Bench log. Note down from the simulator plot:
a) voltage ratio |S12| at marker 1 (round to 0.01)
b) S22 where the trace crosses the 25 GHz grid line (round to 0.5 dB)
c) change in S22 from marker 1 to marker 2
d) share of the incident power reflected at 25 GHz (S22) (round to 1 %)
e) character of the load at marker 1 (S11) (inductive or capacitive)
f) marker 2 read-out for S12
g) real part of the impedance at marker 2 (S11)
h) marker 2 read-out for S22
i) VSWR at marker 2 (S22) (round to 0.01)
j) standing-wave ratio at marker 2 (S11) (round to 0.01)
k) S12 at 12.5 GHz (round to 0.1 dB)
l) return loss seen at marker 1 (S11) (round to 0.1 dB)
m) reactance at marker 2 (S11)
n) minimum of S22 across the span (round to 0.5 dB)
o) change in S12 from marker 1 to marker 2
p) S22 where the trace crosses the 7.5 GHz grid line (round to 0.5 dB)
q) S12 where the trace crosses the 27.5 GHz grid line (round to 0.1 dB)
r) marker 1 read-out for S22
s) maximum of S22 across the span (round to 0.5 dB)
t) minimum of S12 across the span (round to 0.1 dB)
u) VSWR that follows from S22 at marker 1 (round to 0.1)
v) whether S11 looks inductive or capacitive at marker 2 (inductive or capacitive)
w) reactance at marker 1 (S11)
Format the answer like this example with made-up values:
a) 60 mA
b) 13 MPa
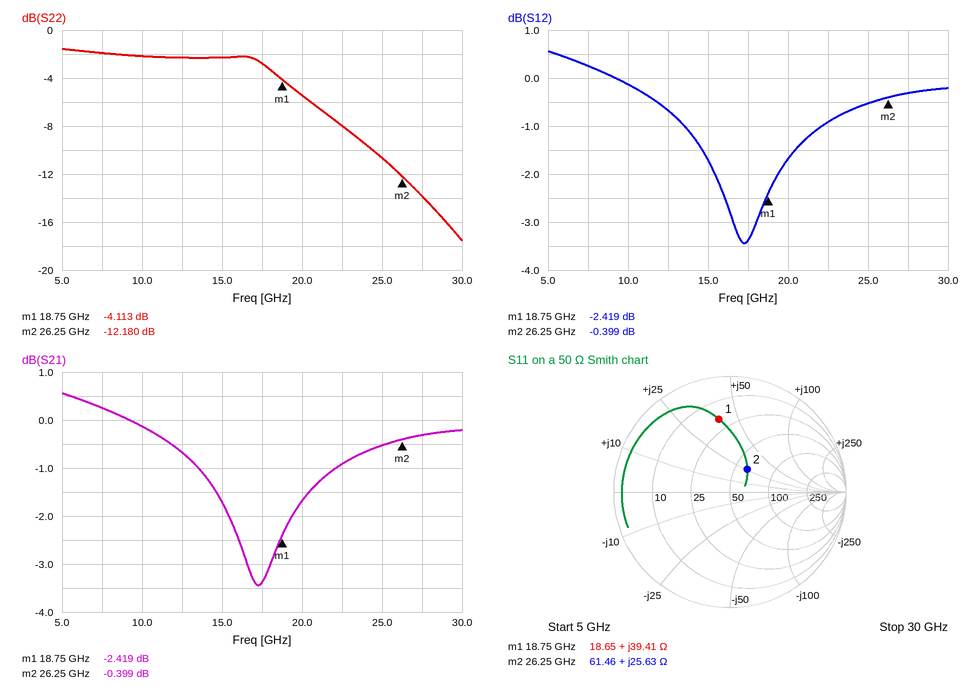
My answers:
a) 0.76
b) -10.5 dB
c) -8.067 dB
d) 9 %
e) inductive
f) -0.399 dB
g) 61.46 Ω
h) -12.180 dB
i) 1.65
j) 1.65
k) -0.7 dB
l) 3.9 dB
m) +25.63 Ω
n) -17.5 dB
o) 2.020 dB
p) -2.0 dB
q) -0.3 dB
r) -4.113 dB
s) -1.5 dB
t) -3.4 dB
u) 4.3
v) inductive
w) +39.41 Ω
